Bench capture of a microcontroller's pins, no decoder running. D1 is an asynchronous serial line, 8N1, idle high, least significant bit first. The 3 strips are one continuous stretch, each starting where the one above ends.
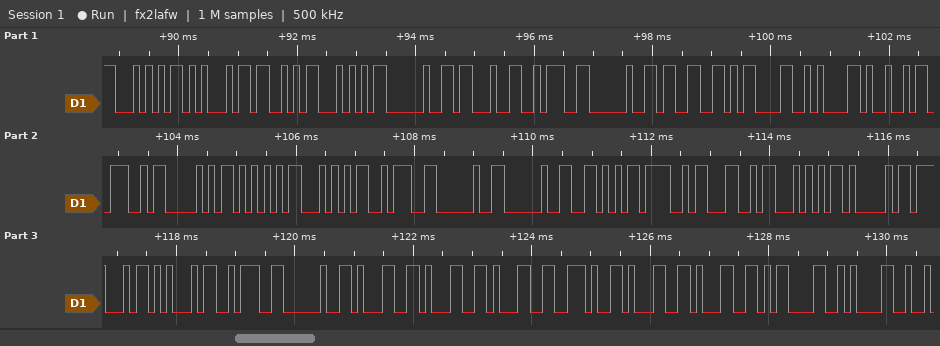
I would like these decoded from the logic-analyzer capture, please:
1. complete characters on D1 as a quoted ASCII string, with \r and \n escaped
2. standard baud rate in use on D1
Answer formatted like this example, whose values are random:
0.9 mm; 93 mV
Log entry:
"TEST #: 3\r\nINPUT:  VOLTAGE: 111.11\r\n"; 9600 baud
